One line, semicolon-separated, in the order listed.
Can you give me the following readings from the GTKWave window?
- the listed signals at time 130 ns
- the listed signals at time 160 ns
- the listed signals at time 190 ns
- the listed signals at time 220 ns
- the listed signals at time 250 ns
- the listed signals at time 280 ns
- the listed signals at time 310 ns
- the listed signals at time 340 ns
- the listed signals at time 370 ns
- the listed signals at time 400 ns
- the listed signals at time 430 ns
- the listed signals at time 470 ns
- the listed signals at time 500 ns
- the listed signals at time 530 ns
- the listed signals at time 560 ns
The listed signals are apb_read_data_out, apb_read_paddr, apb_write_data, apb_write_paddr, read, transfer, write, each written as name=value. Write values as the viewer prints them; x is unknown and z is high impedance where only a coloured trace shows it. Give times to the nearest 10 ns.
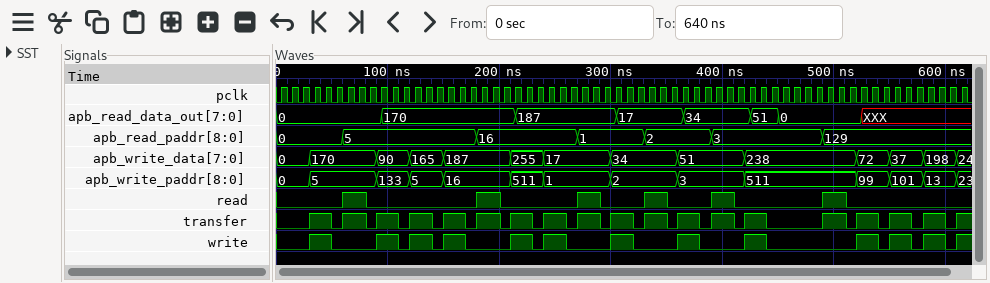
apb_read_data_out=170, apb_read_paddr=5, apb_write_data=165, apb_write_paddr=5, read=0, transfer=1, write=1; apb_read_data_out=170, apb_read_paddr=5, apb_write_data=187, apb_write_paddr=16, read=0, transfer=1, write=1; apb_read_data_out=170, apb_read_paddr=16, apb_write_data=187, apb_write_paddr=16, read=1, transfer=1, write=0; apb_read_data_out=187, apb_read_paddr=16, apb_write_data=255, apb_write_paddr=511, read=0, transfer=1, write=1; apb_read_data_out=187, apb_read_paddr=16, apb_write_data=17, apb_write_paddr=1, read=0, transfer=1, write=1; apb_read_data_out=187, apb_read_paddr=1, apb_write_data=17, apb_write_paddr=1, read=1, transfer=1, write=0; apb_read_data_out=17, apb_read_paddr=1, apb_write_data=34, apb_write_paddr=2, read=0, transfer=1, write=1; apb_read_data_out=17, apb_read_paddr=2, apb_write_data=34, apb_write_paddr=2, read=1, transfer=1, write=0; apb_read_data_out=34, apb_read_paddr=2, apb_write_data=51, apb_write_paddr=3, read=0, transfer=1, write=1; apb_read_data_out=34, apb_read_paddr=3, apb_write_data=51, apb_write_paddr=3, read=1, transfer=1, write=0; apb_read_data_out=51, apb_read_paddr=3, apb_write_data=238, apb_write_paddr=511, read=0, transfer=1, write=1; apb_read_data_out=0, apb_read_paddr=3, apb_write_data=238, apb_write_paddr=511, read=0, transfer=0, write=0; apb_read_data_out=0, apb_read_paddr=129, apb_write_data=238, apb_write_paddr=511, read=1, transfer=1, write=0; apb_read_data_out=XXX, apb_read_paddr=129, apb_write_data=72, apb_write_paddr=99, read=0, transfer=1, write=1; apb_read_data_out=XXX, apb_read_paddr=129, apb_write_data=37, apb_write_paddr=101, read=0, transfer=1, write=1
